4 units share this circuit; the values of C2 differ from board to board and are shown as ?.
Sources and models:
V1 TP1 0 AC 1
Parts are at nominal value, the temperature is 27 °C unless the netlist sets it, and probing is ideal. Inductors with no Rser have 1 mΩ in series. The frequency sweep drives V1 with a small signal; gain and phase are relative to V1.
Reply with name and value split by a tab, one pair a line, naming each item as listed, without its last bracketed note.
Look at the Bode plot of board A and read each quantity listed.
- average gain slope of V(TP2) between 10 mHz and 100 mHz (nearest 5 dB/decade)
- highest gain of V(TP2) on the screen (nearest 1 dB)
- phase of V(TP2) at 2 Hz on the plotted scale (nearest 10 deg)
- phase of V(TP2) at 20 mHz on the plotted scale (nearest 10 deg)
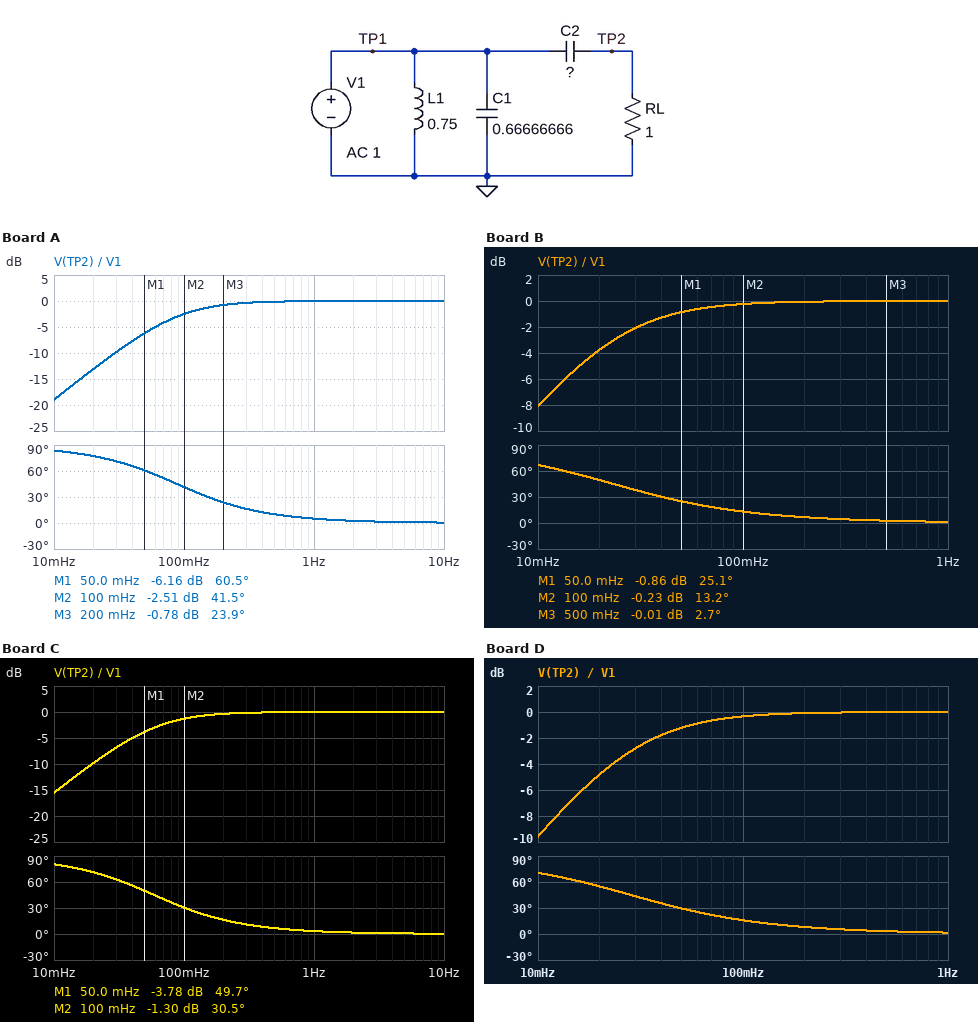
average gain slope of V(TP2) between 10 mHz and 100 mHz	15 dB/decade
highest gain of V(TP2) on the screen	0 dB
phase of V(TP2) at 2 Hz on the plotted scale	0 deg
phase of V(TP2) at 20 mHz on the plotted scale	80 deg
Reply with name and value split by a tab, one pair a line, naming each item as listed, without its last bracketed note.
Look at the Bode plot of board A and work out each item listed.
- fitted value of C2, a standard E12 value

fitted value of C2, a standard E12 value	1.8 F
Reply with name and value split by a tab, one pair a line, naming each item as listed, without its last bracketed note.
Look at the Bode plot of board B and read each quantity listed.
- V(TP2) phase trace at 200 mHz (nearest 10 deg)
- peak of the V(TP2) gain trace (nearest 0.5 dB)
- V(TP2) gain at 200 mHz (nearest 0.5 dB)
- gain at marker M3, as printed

V(TP2) phase trace at 200 mHz	10 deg
peak of the V(TP2) gain trace	0 dB
V(TP2) gain at 200 mHz	0 dB
gain at marker M3, as printed	-0.01 dB
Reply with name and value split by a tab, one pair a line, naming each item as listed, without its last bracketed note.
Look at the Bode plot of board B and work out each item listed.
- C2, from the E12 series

C2, from the E12 series	6.8 F
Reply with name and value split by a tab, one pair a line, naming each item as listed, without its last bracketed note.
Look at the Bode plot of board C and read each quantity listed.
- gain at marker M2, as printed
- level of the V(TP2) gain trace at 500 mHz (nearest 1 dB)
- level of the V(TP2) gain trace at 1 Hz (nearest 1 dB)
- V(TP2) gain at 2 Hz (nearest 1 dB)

gain at marker M2, as printed	-1.30 dB
level of the V(TP2) gain trace at 500 mHz	0 dB
level of the V(TP2) gain trace at 1 Hz	0 dB
V(TP2) gain at 2 Hz	0 dB
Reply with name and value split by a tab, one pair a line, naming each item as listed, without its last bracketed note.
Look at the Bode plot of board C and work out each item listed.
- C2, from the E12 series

C2, from the E12 series	2.7 F
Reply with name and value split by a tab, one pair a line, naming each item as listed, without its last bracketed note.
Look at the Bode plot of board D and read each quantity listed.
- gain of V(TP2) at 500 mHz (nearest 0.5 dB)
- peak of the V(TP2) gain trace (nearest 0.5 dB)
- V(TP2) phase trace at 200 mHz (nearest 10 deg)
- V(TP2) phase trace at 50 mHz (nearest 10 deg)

gain of V(TP2) at 500 mHz	0 dB
peak of the V(TP2) gain trace	0 dB
V(TP2) phase trace at 200 mHz	10 deg
V(TP2) phase trace at 50 mHz	30 deg
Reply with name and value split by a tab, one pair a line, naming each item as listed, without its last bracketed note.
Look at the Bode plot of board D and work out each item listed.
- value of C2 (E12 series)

value of C2	5.6 F
